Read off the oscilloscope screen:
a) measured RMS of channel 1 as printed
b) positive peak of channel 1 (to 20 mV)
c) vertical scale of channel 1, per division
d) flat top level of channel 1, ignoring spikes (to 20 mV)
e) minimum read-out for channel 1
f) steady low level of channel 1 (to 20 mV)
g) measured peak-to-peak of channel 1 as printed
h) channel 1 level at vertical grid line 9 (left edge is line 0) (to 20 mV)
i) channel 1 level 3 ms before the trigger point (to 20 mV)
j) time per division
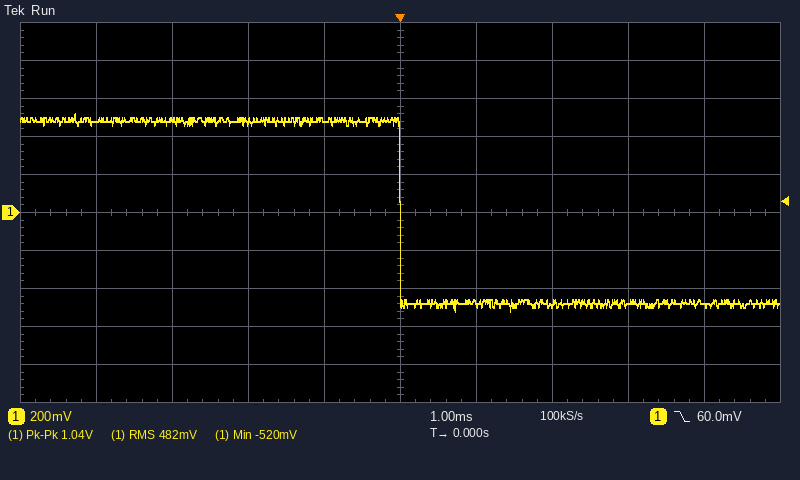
482 mV
520 mV
200 mV
480 mV
-520 mV
-480 mV
1.04 V
-480 mV
480 mV
1 ms
